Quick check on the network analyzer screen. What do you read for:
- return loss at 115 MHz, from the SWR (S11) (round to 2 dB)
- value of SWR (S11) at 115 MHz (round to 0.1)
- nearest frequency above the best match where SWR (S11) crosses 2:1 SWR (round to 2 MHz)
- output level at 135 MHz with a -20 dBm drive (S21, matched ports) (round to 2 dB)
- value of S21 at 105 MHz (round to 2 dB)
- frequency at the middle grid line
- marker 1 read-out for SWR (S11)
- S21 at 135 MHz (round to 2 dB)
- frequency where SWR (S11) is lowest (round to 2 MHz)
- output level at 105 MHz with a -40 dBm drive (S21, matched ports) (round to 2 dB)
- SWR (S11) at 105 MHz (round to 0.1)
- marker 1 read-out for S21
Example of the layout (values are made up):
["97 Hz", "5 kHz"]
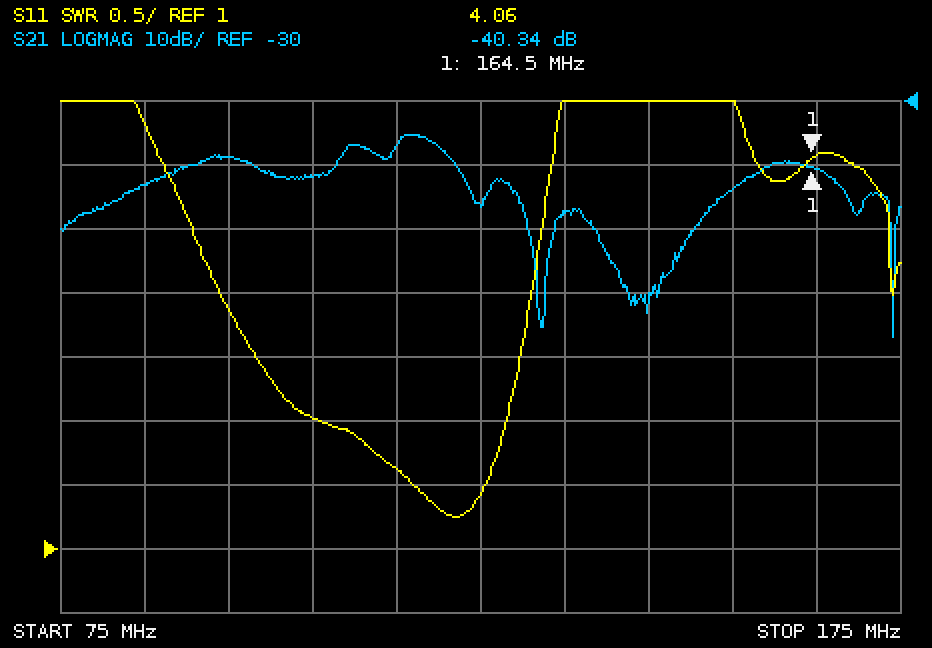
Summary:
["12 dB", "1.6", "128 MHz", "-68 dBm", "-42 dB", "125 MHz", "4.06", "-48 dB", "122 MHz", "-82 dBm", "2.0", "-40.34 dB"]
